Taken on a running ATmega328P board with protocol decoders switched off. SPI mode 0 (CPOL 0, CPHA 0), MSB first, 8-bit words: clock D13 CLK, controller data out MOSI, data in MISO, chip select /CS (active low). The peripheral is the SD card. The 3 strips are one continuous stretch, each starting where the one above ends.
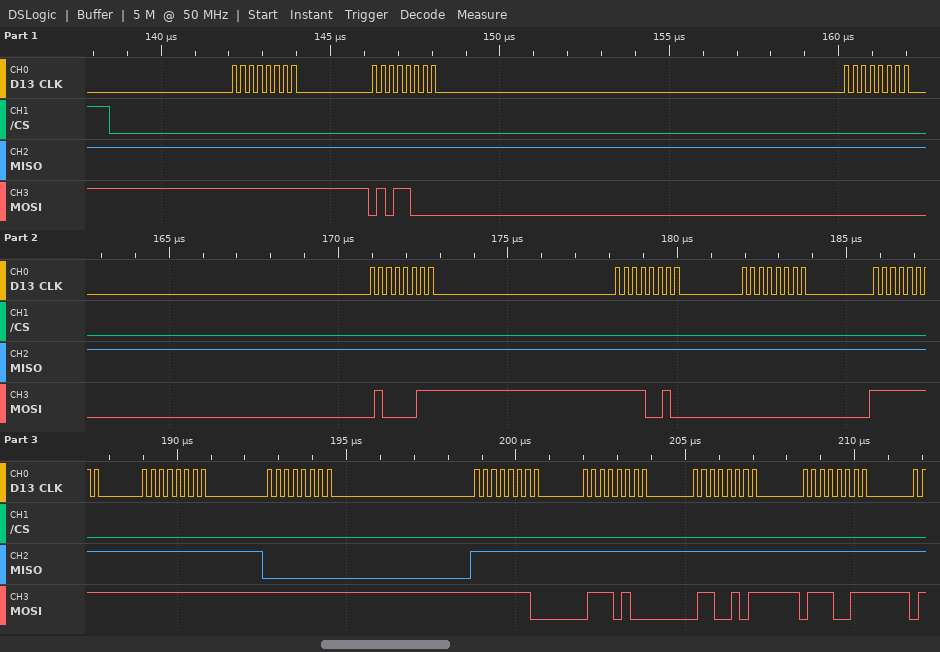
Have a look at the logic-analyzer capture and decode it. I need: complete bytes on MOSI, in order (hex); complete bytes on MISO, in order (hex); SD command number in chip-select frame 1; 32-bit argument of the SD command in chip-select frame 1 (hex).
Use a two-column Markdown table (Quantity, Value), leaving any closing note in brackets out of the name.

| Quantity | Value |
|---|---|
| complete bytes on MOSI, in order | FF 58 00 43 F2 00 FF FF FF FE 74 65 73 |
| complete bytes on MISO, in order | FF FF FF FF FF FF FF FF 00 FF FF FF FF |
| SD command number in chip-select frame 1 | CMD24 |
| 32-bit argument of the SD command in chip-select frame 1 | 0x0043F200 |
